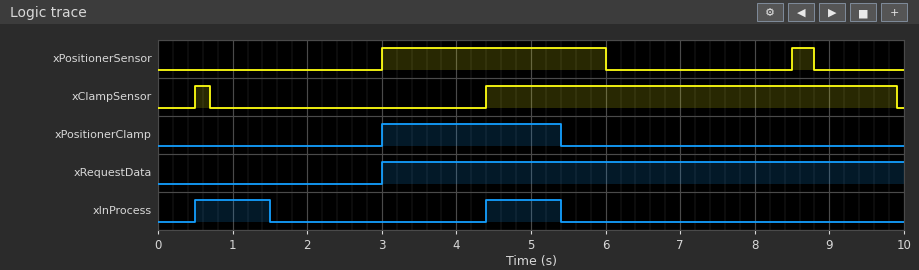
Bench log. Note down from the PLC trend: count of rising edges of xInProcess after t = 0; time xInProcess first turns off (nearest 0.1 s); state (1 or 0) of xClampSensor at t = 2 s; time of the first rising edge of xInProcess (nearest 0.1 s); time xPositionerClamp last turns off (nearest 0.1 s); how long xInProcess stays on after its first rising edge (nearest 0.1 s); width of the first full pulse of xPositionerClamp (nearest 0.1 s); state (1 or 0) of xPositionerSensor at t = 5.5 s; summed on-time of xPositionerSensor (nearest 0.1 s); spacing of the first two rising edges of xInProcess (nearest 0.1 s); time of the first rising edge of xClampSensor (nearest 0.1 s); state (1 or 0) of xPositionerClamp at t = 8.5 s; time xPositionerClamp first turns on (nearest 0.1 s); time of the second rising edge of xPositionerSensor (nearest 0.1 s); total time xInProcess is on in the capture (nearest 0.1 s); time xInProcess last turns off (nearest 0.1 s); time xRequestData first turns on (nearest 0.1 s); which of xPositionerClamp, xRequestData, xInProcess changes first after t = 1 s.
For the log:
2
1.5 s
0
0.5 s
5.4 s
1.0 s
2.4 s
1
3.3 s
3.9 s
0.5 s
0
3.0 s
8.5 s
2.0 s
5.4 s
3.0 s
xInProcess
